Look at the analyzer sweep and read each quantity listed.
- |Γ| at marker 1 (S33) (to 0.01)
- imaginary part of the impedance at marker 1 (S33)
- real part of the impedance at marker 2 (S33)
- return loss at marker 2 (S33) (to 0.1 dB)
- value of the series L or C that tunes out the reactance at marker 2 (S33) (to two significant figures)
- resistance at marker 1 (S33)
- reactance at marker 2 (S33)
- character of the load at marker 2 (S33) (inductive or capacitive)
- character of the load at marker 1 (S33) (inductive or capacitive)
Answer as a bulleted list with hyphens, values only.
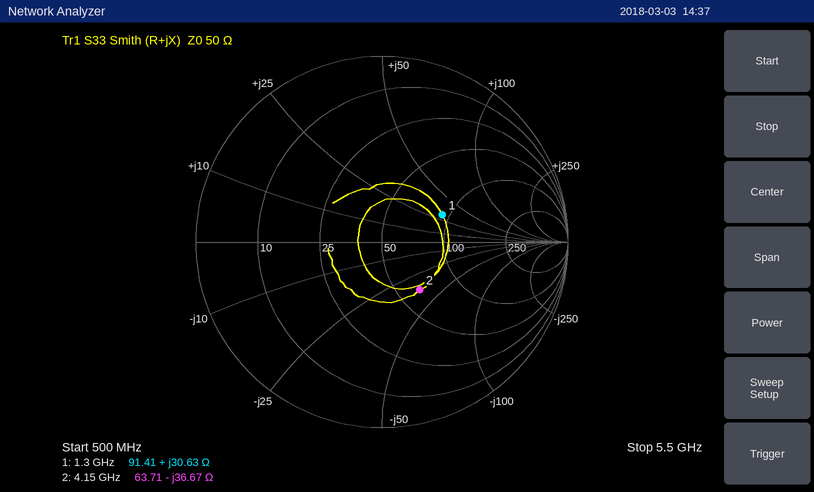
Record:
- 0.36
- +30.63 Ω
- 63.71 Ω
- 9.7 dB
- 1.4 nH
- 91.41 Ω
- -36.67 Ω
- capacitive
- inductive
